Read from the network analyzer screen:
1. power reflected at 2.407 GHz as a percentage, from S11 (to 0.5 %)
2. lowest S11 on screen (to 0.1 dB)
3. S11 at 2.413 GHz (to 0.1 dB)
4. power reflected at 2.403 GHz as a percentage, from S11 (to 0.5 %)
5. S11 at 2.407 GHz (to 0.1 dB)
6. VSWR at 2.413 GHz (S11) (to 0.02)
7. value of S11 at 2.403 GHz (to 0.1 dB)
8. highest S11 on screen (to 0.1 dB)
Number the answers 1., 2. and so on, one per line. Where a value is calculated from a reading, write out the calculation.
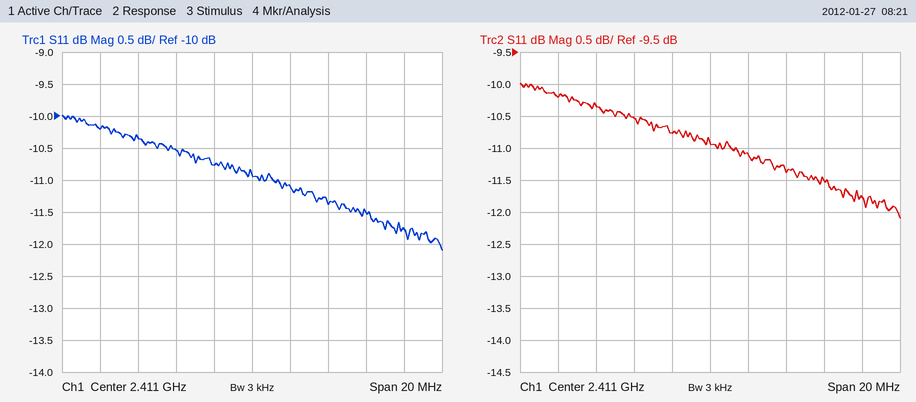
1. 10^(-10.5/10) ≈ 8.91 %, so 9.0 % to the nearest 0.5 %
2. -12.1 dB
3. -11.1 dB
4. 10^(-10.2/10) ≈ 9.5 %
5. -10.5 dB
6. |Γ| = 10^(-11.1/20) = 0.2786; VSWR = (1 + 0.2786)/(1 − 0.2786) ≈ 1.77, so 1.78 to the nearest 0.02
7. -10.2 dB
8. -10.0 dB
